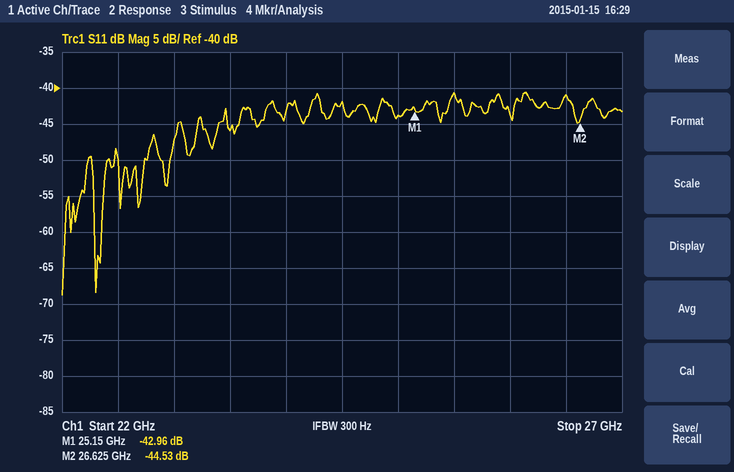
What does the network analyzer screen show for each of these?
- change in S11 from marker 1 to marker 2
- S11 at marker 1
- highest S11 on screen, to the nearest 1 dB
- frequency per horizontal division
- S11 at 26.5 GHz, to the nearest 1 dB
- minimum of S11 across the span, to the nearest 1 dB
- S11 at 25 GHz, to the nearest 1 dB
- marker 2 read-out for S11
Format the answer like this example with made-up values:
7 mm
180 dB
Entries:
-1.57 dB
-42.96 dB
-41 dB
500 MHz
-41 dB
-69 dB
-44 dB
-44.53 dB
